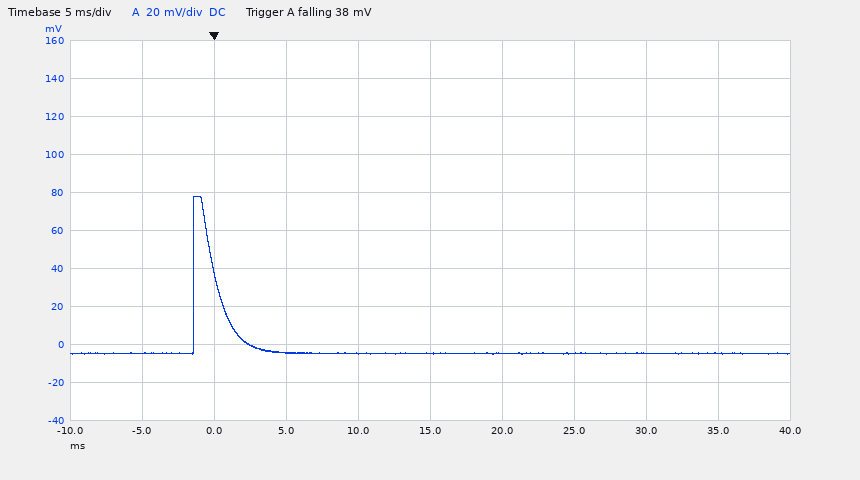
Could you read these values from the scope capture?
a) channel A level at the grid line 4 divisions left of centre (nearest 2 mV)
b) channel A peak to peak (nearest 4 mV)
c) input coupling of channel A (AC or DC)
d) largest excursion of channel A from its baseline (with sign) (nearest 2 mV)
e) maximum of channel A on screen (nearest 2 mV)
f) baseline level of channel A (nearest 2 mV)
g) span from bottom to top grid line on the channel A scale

-4 mV
84 mV
DC
+82 mV
78 mV
-4 mV
200 mV
